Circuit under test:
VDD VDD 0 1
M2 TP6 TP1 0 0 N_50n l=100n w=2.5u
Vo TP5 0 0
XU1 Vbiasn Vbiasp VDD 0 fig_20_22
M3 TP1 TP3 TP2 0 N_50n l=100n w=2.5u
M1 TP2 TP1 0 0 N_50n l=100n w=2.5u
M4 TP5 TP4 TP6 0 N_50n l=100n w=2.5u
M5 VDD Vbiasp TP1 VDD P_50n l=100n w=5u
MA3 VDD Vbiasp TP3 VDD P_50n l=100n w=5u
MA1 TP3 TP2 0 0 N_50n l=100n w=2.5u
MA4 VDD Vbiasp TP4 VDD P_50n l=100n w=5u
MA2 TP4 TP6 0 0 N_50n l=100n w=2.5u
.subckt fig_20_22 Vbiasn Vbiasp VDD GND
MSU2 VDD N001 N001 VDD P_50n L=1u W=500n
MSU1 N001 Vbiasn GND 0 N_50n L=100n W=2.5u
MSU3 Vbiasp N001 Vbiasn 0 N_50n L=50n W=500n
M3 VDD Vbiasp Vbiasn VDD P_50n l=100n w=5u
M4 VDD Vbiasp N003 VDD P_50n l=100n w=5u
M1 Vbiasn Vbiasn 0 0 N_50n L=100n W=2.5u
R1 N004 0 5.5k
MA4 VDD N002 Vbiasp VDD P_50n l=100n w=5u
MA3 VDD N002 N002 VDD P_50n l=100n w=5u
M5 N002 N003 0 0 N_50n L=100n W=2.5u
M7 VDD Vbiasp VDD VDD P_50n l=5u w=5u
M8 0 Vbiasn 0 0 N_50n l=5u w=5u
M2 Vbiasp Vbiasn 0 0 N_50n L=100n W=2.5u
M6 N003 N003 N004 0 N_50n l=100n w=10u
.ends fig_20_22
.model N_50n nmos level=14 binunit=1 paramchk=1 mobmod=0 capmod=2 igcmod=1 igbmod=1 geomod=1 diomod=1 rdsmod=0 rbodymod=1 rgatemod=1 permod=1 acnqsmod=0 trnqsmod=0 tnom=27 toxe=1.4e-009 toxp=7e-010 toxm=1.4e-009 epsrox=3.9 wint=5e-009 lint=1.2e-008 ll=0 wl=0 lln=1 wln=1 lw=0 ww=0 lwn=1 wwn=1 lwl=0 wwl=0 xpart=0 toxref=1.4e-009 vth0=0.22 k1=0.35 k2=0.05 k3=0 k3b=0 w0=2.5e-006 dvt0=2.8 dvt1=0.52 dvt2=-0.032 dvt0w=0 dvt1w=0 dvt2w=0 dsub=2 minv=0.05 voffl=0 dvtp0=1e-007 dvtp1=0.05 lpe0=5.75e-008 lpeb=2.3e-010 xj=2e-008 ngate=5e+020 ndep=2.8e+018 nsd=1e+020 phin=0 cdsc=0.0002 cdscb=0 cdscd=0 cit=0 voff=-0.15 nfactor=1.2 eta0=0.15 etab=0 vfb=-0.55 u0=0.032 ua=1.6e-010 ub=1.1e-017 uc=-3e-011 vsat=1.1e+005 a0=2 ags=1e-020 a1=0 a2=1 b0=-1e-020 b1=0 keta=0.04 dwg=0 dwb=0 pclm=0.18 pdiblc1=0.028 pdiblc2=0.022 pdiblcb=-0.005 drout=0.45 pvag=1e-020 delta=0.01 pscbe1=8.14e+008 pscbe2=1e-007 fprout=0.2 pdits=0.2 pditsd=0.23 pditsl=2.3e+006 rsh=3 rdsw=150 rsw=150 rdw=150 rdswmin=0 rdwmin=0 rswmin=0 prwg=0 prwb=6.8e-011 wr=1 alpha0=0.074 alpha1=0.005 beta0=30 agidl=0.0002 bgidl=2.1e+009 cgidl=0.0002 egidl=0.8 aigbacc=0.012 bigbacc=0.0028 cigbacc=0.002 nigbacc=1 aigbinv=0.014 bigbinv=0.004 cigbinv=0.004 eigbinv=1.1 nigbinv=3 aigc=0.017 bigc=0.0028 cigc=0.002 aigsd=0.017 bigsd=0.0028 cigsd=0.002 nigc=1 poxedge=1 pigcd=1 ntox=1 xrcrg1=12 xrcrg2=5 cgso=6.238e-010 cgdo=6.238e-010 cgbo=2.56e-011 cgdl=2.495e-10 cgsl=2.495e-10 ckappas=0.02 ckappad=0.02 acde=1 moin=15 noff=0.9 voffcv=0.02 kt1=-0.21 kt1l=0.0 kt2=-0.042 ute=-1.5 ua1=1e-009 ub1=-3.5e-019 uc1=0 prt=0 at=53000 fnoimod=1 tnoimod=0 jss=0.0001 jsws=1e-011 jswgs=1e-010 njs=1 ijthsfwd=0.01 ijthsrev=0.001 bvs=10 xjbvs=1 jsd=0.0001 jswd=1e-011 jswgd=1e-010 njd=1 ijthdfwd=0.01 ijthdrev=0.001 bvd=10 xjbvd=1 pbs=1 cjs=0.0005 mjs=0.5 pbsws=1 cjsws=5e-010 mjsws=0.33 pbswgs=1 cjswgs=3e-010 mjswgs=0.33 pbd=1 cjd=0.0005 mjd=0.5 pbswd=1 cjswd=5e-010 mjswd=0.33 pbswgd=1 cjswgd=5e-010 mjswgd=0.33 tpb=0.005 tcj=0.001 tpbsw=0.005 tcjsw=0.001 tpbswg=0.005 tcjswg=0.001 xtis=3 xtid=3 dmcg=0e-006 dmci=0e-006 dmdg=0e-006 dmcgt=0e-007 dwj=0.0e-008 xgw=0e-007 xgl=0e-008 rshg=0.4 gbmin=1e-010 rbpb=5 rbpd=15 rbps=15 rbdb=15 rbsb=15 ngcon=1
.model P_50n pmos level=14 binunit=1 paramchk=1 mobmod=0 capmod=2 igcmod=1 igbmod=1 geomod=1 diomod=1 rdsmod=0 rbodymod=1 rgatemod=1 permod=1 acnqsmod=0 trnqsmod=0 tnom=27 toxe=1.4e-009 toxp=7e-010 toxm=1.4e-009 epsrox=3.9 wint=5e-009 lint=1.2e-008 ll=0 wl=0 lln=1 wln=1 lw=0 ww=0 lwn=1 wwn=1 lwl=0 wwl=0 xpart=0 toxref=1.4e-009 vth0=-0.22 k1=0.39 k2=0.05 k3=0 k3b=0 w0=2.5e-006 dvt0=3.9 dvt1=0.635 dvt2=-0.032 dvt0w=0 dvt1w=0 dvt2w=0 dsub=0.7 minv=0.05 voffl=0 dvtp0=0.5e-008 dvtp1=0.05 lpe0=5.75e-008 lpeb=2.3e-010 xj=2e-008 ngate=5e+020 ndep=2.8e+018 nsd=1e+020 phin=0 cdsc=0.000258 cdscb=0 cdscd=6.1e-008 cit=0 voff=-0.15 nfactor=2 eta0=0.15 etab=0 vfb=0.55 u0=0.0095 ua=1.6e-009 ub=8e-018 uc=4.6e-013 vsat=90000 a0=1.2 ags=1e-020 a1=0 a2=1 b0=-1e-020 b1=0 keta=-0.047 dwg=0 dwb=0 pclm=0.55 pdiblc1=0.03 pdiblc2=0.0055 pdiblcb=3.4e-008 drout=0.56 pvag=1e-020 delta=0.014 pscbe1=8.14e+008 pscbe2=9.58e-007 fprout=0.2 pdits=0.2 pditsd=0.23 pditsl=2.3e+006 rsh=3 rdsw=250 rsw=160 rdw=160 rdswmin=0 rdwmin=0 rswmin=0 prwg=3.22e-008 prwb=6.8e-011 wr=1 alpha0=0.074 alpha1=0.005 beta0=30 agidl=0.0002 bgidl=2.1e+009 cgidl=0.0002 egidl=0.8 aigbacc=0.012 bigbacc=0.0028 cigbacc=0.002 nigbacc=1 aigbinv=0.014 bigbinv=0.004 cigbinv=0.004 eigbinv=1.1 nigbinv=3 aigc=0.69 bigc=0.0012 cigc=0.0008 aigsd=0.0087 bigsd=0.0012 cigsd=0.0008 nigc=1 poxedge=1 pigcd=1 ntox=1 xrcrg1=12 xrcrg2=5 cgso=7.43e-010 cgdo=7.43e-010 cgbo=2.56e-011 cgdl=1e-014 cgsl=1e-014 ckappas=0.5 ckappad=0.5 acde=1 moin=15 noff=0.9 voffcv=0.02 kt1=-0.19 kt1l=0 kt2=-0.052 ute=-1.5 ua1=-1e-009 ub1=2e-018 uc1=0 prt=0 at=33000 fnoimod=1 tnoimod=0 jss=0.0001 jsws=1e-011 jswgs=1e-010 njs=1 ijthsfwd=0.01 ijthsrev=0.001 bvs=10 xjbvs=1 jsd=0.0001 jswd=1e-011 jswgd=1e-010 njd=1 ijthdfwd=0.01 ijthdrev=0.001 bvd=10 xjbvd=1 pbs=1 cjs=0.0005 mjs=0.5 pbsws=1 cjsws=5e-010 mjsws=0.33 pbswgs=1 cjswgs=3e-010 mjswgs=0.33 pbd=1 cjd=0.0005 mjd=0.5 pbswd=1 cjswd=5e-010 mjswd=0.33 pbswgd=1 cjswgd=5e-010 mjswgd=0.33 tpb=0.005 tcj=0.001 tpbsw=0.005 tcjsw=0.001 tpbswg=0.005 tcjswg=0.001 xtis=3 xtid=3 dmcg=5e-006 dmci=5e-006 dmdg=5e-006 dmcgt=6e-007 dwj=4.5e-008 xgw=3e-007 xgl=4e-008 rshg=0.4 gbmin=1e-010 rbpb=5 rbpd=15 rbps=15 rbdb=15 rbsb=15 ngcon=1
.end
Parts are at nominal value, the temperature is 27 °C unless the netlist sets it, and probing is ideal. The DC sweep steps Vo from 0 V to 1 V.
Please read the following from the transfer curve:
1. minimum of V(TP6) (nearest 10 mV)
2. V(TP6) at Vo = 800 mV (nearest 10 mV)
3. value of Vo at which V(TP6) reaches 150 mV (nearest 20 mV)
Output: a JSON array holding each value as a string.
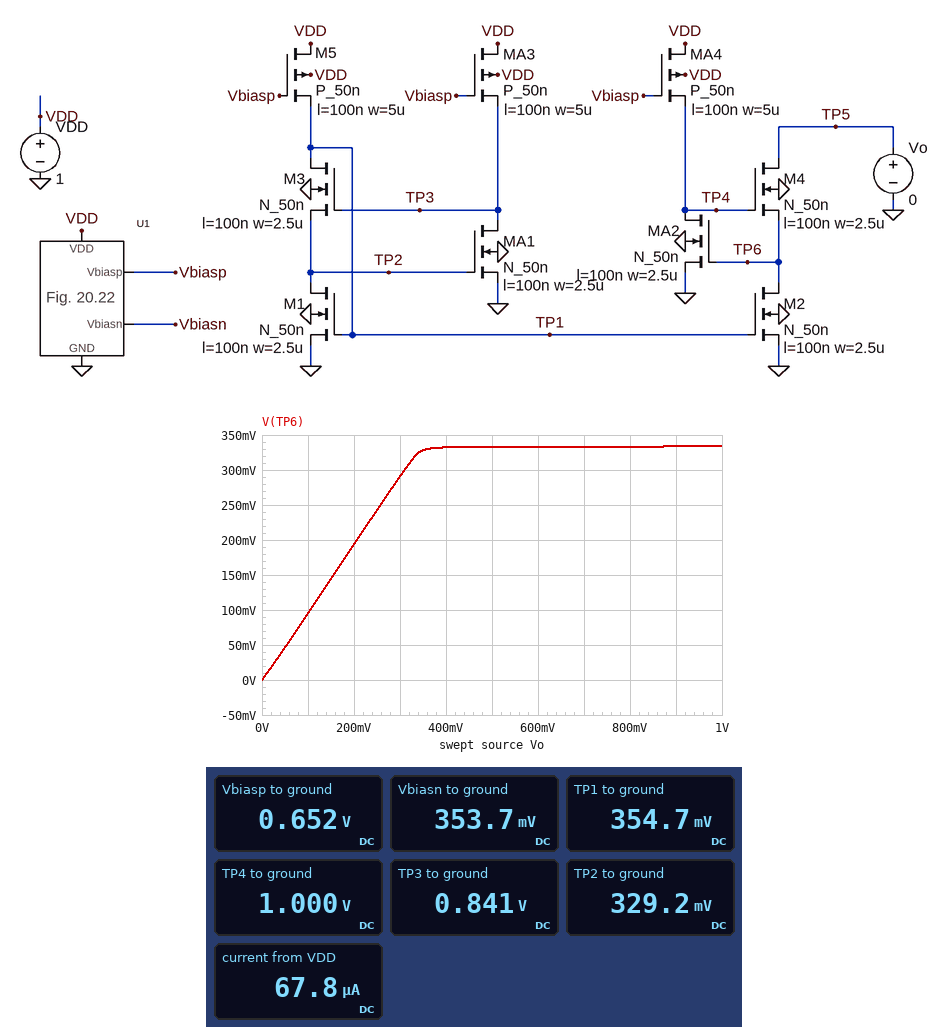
["0 V", "330 mV", "160 mV"]
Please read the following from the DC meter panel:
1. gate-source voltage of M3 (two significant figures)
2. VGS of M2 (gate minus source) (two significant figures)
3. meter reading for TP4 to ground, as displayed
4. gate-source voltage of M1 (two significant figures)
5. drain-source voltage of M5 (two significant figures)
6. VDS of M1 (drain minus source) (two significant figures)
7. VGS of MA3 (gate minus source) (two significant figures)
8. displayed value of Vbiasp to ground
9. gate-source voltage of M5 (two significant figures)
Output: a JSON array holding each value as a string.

["510 mV", "350 mV", "1.000 V", "350 mV", "650 mV", "330 mV", "-190 mV", "0.652 V", "300 mV"]
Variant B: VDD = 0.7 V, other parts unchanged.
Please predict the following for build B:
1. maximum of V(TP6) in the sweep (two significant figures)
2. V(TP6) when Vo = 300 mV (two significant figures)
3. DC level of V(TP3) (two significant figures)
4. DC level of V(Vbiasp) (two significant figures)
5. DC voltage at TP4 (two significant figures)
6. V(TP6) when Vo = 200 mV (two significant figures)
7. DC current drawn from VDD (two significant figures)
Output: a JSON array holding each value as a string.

["270 mV", "250 mV", "690 mV", "350 mV", "700 mV", "180 mV", "54 µA"]
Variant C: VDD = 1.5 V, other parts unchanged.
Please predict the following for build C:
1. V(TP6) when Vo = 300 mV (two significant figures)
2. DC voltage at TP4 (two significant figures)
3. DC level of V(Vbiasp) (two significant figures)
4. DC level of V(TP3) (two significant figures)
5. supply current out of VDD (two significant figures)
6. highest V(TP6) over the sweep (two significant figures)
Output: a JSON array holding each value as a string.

["290 mV", "1.5 V", "1.2 V", "850 mV", "80 µA", "340 mV"]
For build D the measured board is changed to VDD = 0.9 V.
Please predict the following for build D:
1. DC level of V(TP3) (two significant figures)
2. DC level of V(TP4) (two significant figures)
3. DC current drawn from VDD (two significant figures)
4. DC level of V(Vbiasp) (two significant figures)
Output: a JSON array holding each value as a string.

["820 mV", "900 mV", "65 µA", "550 mV"]
